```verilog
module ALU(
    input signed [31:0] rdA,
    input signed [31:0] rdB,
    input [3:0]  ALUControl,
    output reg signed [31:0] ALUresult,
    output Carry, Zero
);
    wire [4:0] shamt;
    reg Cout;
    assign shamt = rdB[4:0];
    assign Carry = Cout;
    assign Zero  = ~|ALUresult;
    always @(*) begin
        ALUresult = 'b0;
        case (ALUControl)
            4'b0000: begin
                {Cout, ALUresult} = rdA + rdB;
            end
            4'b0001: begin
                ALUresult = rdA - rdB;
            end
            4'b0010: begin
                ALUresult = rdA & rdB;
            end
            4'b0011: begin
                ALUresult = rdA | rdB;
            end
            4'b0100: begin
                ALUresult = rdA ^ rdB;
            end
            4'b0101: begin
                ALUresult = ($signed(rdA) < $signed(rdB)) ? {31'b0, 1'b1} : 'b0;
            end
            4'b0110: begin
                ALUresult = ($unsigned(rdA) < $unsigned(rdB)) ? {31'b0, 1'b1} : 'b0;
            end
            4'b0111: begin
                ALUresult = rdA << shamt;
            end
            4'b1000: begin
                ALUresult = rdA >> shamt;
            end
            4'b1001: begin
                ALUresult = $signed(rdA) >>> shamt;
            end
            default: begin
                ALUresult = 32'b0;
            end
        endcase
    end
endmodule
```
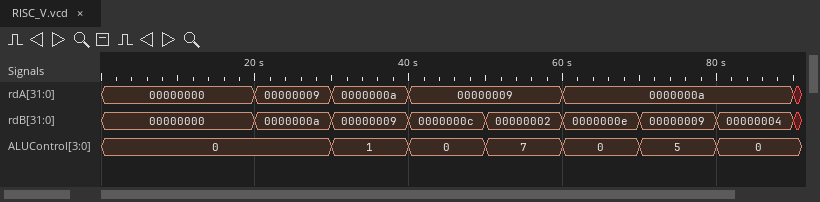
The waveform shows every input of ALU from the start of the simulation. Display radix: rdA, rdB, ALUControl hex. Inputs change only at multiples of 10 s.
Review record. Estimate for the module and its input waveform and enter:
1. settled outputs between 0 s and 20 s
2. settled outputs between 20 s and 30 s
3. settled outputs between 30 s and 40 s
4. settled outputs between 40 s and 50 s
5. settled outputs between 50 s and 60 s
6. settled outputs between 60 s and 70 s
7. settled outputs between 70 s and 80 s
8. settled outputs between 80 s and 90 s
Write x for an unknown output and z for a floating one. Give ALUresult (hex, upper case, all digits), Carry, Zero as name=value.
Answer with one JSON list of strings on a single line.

["ALUresult=00000000, Carry=0, Zero=1", "ALUresult=00000013, Carry=0, Zero=0", "ALUresult=00000001, Carry=0, Zero=0", "ALUresult=00000015, Carry=0, Zero=0", "ALUresult=00000024, Carry=0, Zero=0", "ALUresult=00000018, Carry=0, Zero=0", "ALUresult=00000000, Carry=0, Zero=1", "ALUresult=0000000E, Carry=0, Zero=0"]
